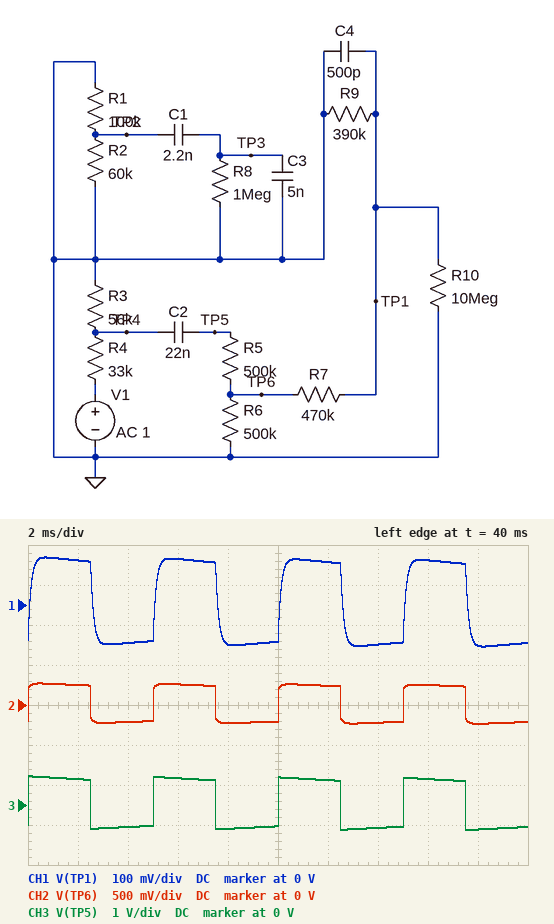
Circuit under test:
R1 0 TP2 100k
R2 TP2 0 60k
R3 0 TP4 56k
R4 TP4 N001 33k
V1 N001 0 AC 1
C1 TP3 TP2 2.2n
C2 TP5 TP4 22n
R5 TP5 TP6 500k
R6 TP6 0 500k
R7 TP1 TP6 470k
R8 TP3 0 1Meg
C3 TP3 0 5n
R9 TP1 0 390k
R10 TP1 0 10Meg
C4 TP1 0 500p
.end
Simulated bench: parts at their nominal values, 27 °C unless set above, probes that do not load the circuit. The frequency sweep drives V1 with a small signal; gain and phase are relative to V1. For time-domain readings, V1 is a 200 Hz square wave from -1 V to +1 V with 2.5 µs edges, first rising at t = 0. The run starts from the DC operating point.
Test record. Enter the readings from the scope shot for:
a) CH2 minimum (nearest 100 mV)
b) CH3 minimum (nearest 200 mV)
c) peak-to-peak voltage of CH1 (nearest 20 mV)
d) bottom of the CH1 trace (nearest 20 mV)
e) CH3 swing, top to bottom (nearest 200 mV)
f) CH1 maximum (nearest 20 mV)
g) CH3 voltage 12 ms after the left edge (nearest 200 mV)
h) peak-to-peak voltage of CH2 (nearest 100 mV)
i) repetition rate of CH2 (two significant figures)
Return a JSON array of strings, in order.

["-200 mV", "-600 mV", "220 mV", "-100 mV", "1.4 V", "120 mV", "600 mV", "500 mV", "200 Hz"]
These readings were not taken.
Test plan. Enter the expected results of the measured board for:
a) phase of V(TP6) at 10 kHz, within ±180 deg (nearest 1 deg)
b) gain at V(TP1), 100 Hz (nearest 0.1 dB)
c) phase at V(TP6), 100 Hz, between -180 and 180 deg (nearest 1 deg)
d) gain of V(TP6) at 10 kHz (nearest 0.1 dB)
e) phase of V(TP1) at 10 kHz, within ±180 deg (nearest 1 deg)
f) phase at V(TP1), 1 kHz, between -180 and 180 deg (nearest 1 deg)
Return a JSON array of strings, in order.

["-1 deg", "-19.6 dB", "4 deg", "-14.0 dB", "-83 deg", "-37 deg"]
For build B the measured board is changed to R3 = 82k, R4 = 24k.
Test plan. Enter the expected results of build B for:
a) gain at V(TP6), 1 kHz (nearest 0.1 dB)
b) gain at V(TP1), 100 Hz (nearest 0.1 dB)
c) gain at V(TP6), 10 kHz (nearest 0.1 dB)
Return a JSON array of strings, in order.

["-11.2 dB", "-17.8 dB", "-12.1 dB"]
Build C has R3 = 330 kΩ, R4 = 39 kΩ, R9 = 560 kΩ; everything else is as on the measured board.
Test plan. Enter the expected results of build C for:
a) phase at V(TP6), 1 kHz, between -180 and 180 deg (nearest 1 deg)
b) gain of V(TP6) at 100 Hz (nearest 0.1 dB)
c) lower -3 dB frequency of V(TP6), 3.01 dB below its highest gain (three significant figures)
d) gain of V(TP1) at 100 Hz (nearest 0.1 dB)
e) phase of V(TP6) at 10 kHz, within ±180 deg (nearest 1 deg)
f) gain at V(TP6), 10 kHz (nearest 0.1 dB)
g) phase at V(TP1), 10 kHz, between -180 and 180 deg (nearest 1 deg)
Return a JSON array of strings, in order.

["-5 deg", "-9.3 dB", "8.25 Hz", "-14.9 dB", "-1 deg", "-11.1 dB", "-84 deg"]
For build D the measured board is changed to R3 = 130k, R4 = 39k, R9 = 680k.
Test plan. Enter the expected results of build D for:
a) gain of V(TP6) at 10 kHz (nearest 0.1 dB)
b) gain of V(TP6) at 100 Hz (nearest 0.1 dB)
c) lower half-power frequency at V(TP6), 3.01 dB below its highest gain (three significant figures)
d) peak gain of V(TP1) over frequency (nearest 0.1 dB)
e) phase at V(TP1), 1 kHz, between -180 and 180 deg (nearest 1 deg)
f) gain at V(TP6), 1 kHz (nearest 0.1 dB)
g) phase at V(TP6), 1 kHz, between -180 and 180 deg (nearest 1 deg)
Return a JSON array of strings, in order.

["-12.3 dB", "-10.4 dB", "8.18 Hz", "-15.3 dB", "-46 deg", "-11.3 dB", "-6 deg"]
